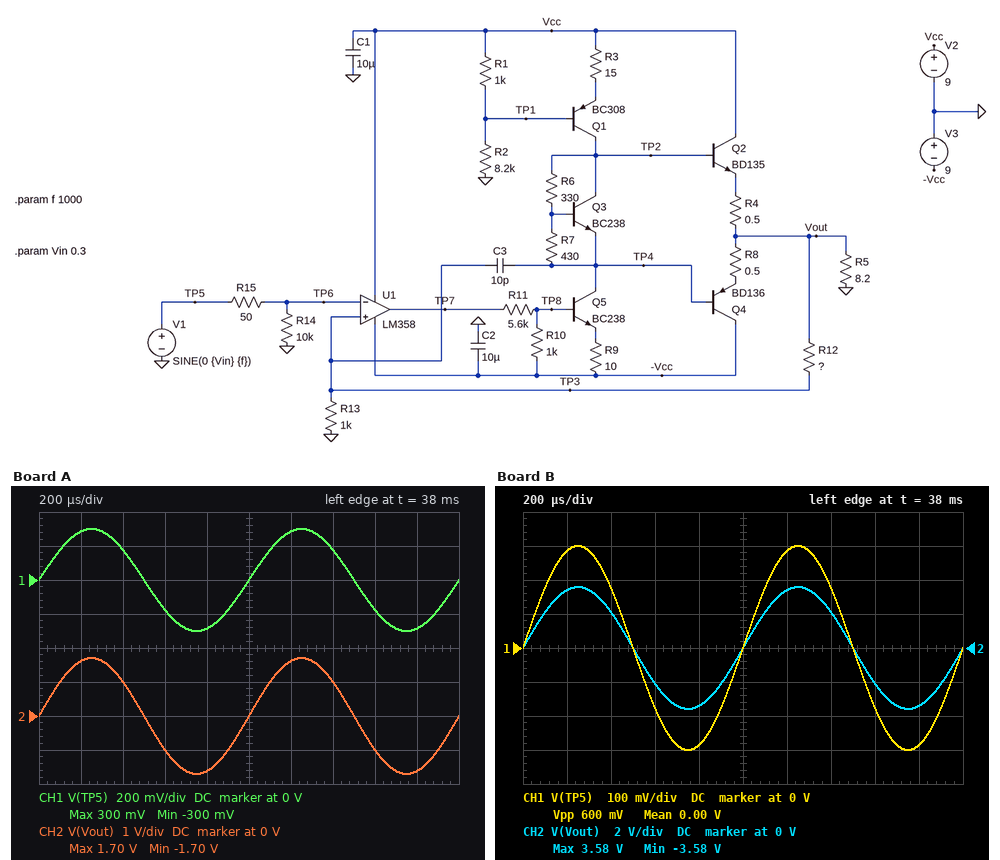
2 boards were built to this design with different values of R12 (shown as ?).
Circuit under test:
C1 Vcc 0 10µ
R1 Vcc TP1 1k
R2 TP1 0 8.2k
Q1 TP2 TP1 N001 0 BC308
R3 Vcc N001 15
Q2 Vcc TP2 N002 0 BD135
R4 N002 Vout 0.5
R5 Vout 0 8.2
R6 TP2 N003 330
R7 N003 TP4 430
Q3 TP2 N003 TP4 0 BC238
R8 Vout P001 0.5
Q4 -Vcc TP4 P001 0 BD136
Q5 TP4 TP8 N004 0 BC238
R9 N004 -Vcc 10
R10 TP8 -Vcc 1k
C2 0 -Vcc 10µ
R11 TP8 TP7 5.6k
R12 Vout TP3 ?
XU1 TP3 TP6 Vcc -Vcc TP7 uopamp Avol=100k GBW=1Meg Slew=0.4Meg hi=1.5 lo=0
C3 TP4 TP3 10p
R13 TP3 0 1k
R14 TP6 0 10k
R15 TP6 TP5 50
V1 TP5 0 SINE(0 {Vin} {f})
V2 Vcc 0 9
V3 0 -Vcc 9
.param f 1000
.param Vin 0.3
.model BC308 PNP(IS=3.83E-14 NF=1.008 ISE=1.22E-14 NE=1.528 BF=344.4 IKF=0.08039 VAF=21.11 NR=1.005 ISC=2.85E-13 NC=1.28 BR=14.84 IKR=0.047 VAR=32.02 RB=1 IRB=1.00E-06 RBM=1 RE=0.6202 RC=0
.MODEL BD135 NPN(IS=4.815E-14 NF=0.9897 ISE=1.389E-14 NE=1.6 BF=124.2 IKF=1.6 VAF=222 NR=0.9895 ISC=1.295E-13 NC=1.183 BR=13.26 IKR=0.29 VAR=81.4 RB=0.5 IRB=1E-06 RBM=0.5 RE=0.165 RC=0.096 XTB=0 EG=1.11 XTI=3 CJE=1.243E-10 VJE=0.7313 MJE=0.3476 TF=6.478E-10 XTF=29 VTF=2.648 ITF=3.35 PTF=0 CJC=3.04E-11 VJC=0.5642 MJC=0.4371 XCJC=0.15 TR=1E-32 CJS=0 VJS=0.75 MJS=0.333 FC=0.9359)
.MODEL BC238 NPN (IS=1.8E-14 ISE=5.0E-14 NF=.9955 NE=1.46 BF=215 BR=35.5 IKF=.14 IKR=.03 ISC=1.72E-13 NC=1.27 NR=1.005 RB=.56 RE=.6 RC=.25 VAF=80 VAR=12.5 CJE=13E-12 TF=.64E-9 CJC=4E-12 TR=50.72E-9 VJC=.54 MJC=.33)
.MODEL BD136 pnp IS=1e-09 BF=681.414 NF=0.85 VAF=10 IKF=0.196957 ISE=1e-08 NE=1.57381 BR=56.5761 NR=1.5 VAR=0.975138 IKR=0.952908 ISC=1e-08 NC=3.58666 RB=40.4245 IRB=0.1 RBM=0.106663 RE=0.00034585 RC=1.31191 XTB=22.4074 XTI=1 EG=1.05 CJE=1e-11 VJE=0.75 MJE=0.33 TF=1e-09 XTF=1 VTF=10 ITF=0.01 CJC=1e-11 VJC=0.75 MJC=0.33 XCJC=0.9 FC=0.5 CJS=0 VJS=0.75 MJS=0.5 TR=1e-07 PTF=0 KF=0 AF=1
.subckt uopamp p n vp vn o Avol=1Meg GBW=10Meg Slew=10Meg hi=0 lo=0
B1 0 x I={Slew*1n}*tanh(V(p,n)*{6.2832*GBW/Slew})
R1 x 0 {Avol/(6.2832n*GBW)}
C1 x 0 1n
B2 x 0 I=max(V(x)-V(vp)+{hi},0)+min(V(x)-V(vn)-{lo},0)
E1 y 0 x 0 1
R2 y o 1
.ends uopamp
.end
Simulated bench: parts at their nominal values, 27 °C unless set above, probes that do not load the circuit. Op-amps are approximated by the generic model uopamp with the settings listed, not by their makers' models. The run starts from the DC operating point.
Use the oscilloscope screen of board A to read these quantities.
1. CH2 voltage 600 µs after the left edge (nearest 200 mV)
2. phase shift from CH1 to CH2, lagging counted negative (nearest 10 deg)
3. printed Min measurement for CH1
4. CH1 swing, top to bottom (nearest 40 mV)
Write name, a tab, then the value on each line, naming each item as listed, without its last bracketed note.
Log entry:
CH2 voltage 600 µs after the left edge	-1.0 V
phase shift from CH1 to CH2, lagging counted negative	0 deg
printed Min measurement for CH1	-300 mV
CH1 swing, top to bottom	600 mV
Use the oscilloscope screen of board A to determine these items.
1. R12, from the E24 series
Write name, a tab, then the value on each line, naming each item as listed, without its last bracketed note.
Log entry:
R12, from the E24 series	4.7 kΩ
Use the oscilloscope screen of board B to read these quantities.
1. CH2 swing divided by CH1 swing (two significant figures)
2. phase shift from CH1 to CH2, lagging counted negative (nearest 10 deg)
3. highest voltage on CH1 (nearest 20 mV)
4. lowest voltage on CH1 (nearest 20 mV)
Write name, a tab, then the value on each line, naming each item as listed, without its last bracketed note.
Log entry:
CH2 swing divided by CH1 swing	12
phase shift from CH1 to CH2, lagging counted negative	0 deg
highest voltage on CH1	300 mV
lowest voltage on CH1	-300 mV
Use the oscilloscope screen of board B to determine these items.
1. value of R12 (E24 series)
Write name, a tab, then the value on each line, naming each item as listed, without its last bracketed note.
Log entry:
value of R12	11 kΩ
